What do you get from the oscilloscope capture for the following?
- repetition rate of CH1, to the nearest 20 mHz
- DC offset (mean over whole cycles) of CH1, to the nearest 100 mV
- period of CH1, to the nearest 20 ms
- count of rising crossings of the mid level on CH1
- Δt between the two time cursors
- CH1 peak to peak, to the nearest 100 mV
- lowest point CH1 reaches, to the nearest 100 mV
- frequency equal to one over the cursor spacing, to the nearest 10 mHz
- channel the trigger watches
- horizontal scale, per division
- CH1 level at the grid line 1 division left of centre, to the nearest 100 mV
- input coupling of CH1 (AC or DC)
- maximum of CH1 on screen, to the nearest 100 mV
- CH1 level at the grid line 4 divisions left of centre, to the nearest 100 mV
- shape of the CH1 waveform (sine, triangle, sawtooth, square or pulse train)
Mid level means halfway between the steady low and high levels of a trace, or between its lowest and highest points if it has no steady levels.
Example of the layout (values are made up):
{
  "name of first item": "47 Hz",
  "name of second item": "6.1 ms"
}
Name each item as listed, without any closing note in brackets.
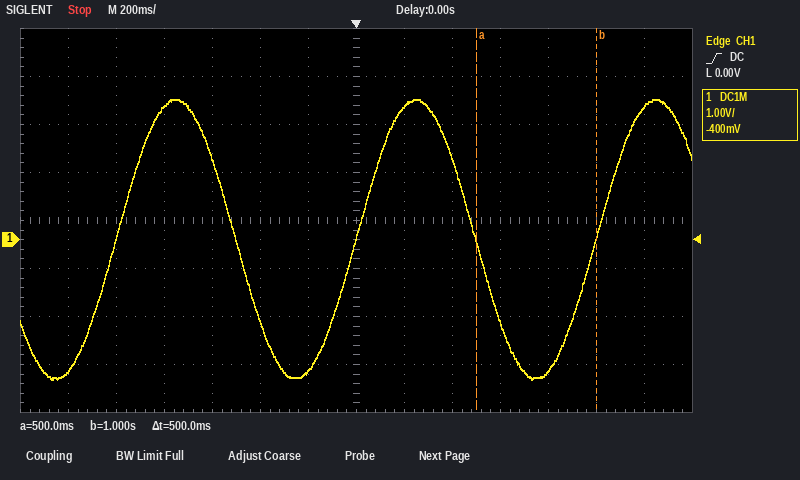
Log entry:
{
  "repetition rate of CH1, to the nearest 20 mHz": "1.00 Hz",
  "DC offset (mean over whole cycles) of CH1, to the nearest 100 mV": "0.0 V",
  "period of CH1, to the nearest 20 ms": "1.00 s",
  "count of rising crossings of the mid level on CH1": "3",
  "Δt between the two time cursors": "500 ms",
  "CH1 peak to peak, to the nearest 100 mV": "5.8 V",
  "lowest point CH1 reaches, to the nearest 100 mV": "-2.9 V",
  "frequency equal to one over the cursor spacing, to the nearest 10 mHz": "2.00 Hz",
  "channel the trigger watches": "CH1",
  "horizontal scale, per division": "200 ms",
  "CH1 level at the grid line 1 division left of centre, to the nearest 100 mV": "-2.7 V",
  "input coupling of CH1": "DC",
  "maximum of CH1 on screen, to the nearest 100 mV": "2.9 V",
  "CH1 level at the grid line 4 divisions left of centre, to the nearest 100 mV": "2.8 V",
  "shape of the CH1 waveform": "sine"
}
